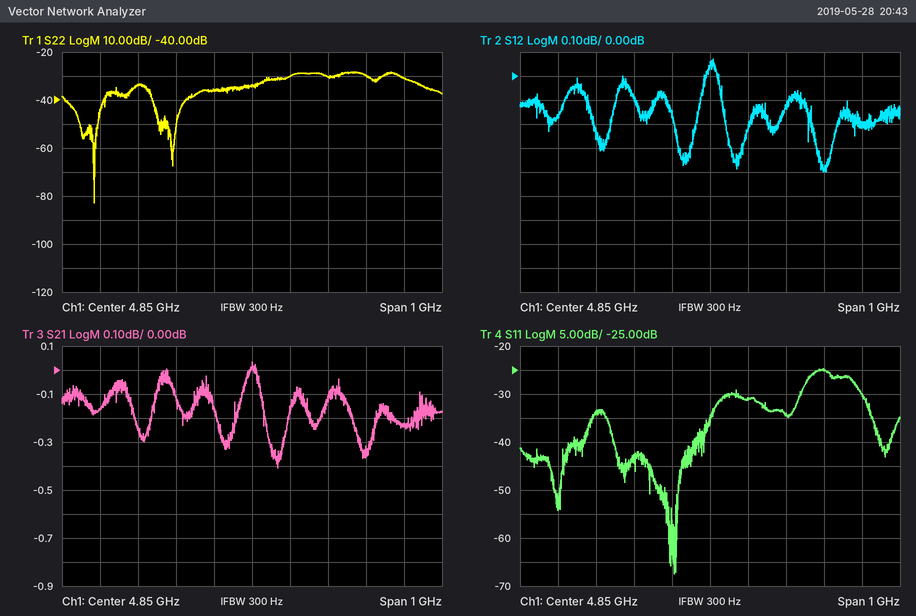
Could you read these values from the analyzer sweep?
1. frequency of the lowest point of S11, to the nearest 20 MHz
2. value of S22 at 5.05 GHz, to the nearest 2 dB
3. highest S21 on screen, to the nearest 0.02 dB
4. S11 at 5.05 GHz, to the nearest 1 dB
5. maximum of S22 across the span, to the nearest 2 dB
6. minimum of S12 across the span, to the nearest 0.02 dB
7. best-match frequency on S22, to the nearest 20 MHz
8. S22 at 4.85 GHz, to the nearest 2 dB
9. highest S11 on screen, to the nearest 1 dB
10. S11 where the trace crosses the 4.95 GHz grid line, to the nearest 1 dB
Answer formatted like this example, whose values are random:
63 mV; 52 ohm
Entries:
4.76 GHz; -30 dB; 0.04 dB; -34 dB; -28 dB; -0.40 dB; 4.44 GHz; -34 dB; -25 dB; -31 dB
